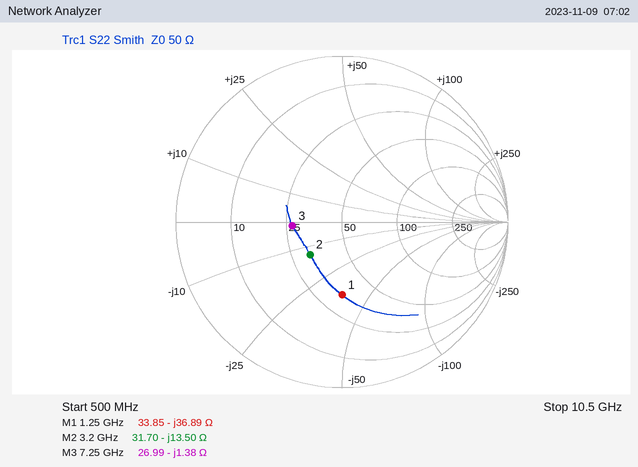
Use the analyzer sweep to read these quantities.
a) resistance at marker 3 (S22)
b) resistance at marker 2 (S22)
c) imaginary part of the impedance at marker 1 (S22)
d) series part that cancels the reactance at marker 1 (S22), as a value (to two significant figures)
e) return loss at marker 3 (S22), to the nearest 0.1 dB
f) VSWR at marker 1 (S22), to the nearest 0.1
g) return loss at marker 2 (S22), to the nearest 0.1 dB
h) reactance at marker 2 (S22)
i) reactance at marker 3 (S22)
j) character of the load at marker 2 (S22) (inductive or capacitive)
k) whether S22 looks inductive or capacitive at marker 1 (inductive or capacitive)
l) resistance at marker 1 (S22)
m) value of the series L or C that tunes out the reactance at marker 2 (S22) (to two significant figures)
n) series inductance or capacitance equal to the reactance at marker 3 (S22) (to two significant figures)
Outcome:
26.99 Ω
31.70 Ω
-36.89 Ω
4.7 nH
10.5 dB
2.6
11.2 dB
-13.50 Ω
-1.38 Ω
capacitive
capacitive
33.85 Ω
670 pH
16 pF
